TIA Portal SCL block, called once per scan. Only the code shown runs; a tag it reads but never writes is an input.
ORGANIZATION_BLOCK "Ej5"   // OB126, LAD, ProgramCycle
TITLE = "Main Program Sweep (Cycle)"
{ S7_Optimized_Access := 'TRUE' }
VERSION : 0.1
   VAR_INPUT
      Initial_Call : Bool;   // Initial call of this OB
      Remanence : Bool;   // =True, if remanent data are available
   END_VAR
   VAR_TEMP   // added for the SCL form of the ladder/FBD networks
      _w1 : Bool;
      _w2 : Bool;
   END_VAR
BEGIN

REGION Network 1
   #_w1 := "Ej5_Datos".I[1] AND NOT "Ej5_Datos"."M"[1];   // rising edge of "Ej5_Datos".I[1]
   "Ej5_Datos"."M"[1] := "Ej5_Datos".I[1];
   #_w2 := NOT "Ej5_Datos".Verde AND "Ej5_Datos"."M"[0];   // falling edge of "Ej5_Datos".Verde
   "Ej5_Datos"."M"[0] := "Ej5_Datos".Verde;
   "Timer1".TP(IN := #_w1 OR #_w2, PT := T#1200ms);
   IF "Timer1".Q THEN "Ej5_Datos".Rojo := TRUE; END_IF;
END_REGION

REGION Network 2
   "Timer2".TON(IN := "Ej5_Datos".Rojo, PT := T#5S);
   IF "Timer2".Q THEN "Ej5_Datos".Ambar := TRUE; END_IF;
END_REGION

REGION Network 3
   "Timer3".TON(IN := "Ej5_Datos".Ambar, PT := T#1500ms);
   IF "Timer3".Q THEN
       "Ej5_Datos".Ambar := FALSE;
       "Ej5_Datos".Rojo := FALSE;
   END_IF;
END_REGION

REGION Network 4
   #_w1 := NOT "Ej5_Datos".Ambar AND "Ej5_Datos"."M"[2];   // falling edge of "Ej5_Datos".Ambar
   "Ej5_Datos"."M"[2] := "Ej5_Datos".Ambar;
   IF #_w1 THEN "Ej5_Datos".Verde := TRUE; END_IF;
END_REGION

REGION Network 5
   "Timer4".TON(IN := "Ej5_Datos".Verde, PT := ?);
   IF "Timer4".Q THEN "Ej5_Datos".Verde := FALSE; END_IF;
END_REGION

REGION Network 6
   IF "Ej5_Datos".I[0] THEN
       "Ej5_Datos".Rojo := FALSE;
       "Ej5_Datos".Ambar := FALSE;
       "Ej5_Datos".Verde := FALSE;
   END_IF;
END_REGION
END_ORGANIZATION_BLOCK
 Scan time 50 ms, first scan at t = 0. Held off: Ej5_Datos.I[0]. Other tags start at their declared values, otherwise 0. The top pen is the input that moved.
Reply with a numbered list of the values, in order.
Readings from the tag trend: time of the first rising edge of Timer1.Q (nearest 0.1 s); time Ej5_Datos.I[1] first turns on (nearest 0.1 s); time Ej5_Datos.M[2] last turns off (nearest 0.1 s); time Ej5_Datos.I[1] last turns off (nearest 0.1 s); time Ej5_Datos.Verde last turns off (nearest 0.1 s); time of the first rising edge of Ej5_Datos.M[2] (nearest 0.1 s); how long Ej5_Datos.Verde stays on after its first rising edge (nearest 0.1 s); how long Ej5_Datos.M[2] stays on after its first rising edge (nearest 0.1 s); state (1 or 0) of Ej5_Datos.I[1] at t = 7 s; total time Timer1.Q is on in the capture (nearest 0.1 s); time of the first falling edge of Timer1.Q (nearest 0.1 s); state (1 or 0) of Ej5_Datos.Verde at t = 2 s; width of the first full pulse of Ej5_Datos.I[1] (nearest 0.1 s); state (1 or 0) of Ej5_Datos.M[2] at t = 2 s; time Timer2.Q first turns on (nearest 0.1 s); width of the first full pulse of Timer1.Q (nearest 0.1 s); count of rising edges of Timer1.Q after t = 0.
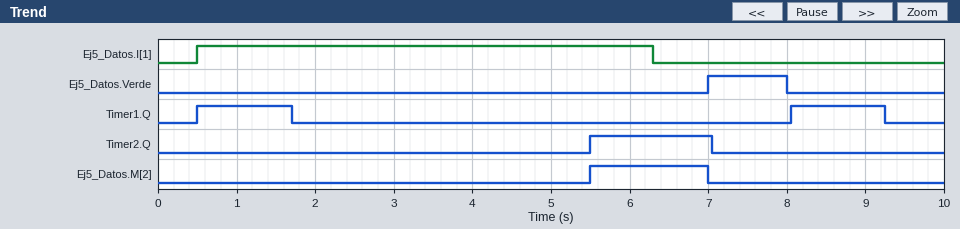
1. 0.5 s
2. 0.5 s
3. 7.0 s
4. 6.3 s
5. 8.0 s
6. 5.5 s
7. 1.0 s
8. 1.5 s
9. 0
10. 2.4 s
11. 1.7 s
12. 0
13. 5.8 s
14. 0
15. 5.5 s
16. 1.2 s
17. 2
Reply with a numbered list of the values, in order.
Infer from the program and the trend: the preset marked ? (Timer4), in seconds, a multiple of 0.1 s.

1. 1.0 s
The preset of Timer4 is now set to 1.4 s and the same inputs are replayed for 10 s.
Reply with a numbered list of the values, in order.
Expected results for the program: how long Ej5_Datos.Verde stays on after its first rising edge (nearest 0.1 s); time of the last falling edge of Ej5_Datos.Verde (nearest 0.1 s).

1. 1.4 s
2. 8.4 s
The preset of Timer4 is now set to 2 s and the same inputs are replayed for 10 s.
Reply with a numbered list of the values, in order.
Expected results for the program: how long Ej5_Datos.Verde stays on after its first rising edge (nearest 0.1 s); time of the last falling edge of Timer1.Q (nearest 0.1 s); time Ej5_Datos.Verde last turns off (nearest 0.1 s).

1. 2.0 s
2. 1.7 s
3. 9.0 s
